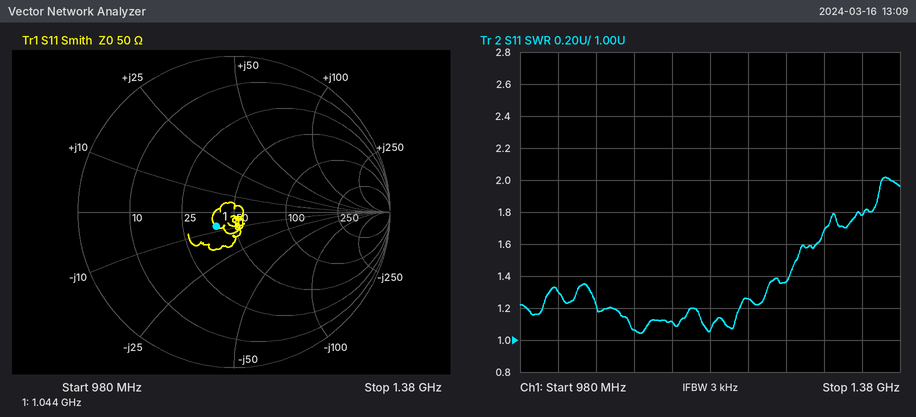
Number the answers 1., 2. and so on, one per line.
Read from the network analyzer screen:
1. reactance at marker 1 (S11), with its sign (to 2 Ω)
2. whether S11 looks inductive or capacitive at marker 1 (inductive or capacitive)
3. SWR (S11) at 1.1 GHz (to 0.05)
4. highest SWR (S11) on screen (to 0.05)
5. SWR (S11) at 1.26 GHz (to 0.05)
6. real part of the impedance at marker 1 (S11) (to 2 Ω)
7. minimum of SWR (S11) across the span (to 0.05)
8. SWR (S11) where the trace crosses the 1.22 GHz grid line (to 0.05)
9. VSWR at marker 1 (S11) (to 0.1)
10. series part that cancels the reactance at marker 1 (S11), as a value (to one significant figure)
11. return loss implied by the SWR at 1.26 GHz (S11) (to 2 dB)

1. -8 Ω
2. capacitive
3. 1.05
4. 2.00
5. 1.35
6. 40 Ω
7. 1.05
8. 1.25
9. 1.3
10. 1 nH
11. 16 dB
